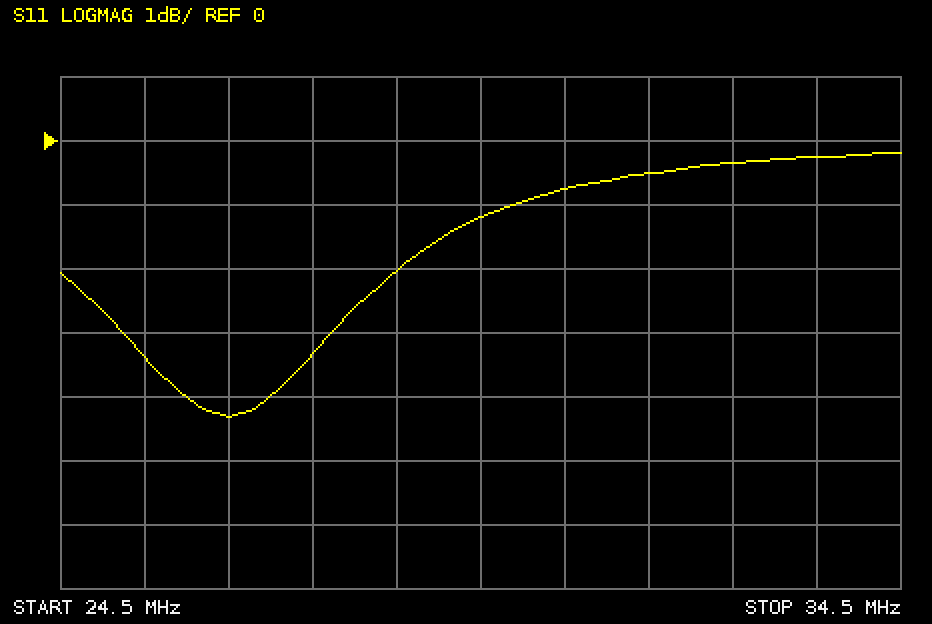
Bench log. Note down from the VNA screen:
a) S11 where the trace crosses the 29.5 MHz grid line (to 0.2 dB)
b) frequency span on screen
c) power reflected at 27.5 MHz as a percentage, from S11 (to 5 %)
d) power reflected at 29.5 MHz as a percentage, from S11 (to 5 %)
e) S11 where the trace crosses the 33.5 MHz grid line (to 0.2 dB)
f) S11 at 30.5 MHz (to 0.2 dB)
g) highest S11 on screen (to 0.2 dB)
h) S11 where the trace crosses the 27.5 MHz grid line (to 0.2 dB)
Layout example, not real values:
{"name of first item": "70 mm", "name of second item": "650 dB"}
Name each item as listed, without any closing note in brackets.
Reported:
{"S11 where the trace crosses the 29.5 MHz grid line": "-1.2 dB", "frequency span on screen": "10 MHz", "power reflected at 27.5 MHz as a percentage, from S11": "45 %", "power reflected at 29.5 MHz as a percentage, from S11": "75 %", "S11 where the trace crosses the 33.5 MHz grid line": "-0.2 dB", "S11 at 30.5 MHz": "-0.8 dB", "highest S11 on screen": "-0.2 dB", "S11 where the trace crosses the 27.5 MHz grid line": "-3.4 dB"}
